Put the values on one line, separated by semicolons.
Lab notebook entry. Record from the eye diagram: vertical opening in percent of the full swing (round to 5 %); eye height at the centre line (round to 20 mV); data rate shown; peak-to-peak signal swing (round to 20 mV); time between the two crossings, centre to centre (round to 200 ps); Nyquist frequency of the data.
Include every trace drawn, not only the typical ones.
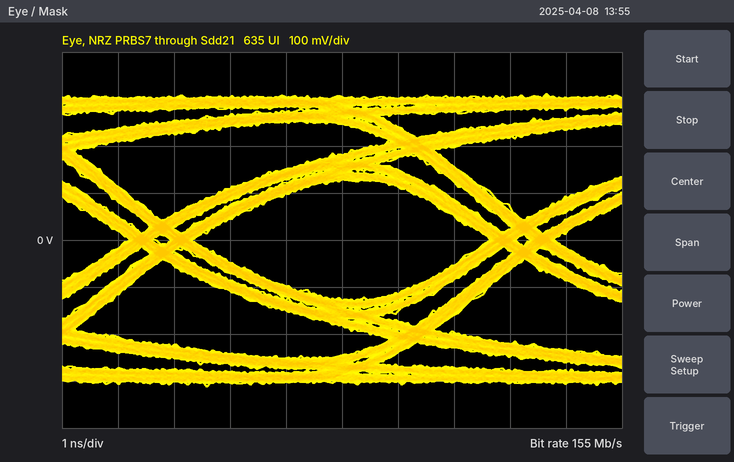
40 %; 260 mV; 155 Mb/s; 620 mV; 6.4 ns; 77.5 MHz
